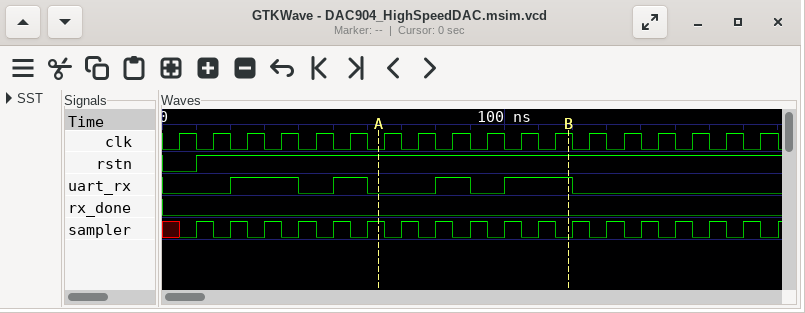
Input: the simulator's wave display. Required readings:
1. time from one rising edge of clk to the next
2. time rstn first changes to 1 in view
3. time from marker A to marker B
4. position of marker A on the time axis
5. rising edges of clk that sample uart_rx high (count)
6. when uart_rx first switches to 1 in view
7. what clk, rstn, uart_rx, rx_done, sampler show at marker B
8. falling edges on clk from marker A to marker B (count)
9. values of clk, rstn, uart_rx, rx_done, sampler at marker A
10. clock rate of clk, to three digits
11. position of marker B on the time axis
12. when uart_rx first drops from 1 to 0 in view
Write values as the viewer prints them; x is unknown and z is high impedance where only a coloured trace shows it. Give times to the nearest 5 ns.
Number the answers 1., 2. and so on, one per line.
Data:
1. 10 ns
2. 10 ns
3. 55 ns
4. 65 ns
5. 6
6. 20 ns
7. clk=1, rstn=1, uart_rx=1, rx_done=0, sampler=0
8. 5
9. clk=0, rstn=1, uart_rx=0, rx_done=0, sampler=1
10. 100 MHz
11. 120 ns
12. 40 ns
